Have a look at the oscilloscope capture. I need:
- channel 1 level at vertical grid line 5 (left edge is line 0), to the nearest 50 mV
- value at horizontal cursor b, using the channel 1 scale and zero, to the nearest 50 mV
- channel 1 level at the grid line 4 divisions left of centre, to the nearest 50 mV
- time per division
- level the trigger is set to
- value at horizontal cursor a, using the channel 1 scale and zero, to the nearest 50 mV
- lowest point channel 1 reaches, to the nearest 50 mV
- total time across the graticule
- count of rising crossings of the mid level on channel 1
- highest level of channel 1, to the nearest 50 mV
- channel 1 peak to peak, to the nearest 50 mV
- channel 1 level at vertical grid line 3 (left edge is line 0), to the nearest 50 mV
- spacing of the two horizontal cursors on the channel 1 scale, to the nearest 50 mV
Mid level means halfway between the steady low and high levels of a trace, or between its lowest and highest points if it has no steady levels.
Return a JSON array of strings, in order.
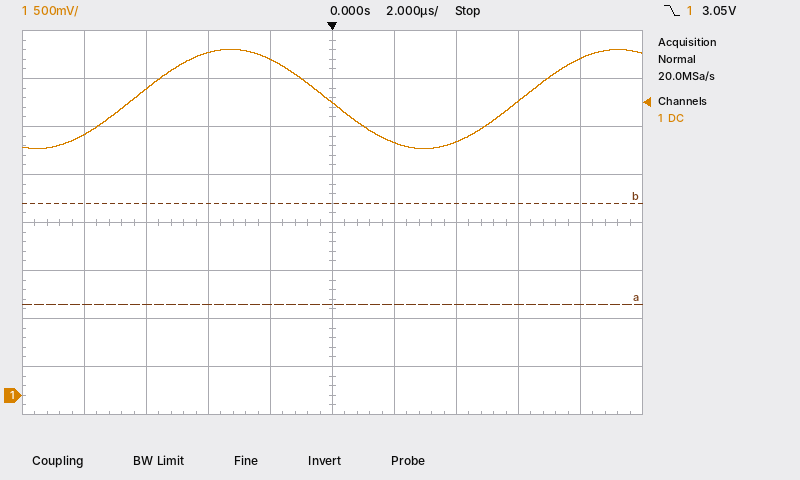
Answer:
["3.05 V", "2.00 V", "2.70 V", "2 µs", "3.05 V", "950 mV", "2.55 V", "20 µs", "2", "3.60 V", "1.05 V", "3.55 V", "1.05 V"]
